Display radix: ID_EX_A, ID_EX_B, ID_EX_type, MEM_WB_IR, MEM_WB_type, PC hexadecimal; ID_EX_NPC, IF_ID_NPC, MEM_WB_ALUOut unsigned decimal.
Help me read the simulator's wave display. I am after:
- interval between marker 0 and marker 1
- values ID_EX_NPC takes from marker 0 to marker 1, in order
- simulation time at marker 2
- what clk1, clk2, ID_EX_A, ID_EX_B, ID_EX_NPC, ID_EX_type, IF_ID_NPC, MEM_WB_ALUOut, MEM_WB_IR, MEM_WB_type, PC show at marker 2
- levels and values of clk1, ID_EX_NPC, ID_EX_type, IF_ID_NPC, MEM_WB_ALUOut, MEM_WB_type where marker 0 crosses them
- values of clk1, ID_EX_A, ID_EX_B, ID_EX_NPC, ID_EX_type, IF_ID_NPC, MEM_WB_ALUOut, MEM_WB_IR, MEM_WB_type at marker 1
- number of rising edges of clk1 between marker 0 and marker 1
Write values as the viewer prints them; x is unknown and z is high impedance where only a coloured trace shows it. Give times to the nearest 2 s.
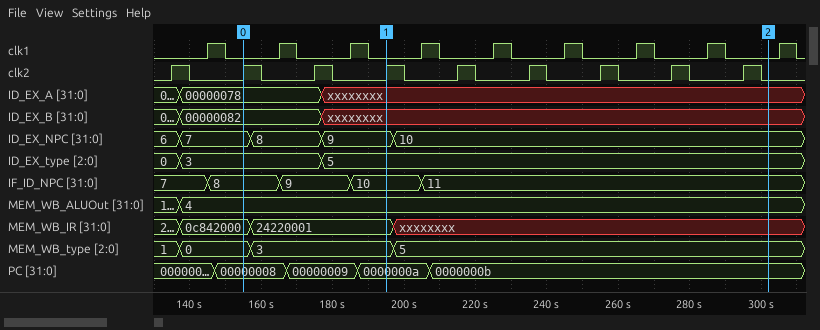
40 s
7, 8, 9
302 s
clk1=0, clk2=0, ID_EX_A=xxxxxxxx, ID_EX_B=xxxxxxxx, ID_EX_NPC=10, ID_EX_type=5, IF_ID_NPC=11, MEM_WB_ALUOut=4, MEM_WB_IR=xxxxxxxx, MEM_WB_type=5, PC=0000000b
clk1=0, ID_EX_NPC=7, ID_EX_type=3, IF_ID_NPC=8, MEM_WB_ALUOut=4, MEM_WB_type=0
clk1=0, ID_EX_A=xxxxxxxx, ID_EX_B=xxxxxxxx, ID_EX_NPC=9, ID_EX_type=5, IF_ID_NPC=10, MEM_WB_ALUOut=4, MEM_WB_IR=24220001, MEM_WB_type=3
2
